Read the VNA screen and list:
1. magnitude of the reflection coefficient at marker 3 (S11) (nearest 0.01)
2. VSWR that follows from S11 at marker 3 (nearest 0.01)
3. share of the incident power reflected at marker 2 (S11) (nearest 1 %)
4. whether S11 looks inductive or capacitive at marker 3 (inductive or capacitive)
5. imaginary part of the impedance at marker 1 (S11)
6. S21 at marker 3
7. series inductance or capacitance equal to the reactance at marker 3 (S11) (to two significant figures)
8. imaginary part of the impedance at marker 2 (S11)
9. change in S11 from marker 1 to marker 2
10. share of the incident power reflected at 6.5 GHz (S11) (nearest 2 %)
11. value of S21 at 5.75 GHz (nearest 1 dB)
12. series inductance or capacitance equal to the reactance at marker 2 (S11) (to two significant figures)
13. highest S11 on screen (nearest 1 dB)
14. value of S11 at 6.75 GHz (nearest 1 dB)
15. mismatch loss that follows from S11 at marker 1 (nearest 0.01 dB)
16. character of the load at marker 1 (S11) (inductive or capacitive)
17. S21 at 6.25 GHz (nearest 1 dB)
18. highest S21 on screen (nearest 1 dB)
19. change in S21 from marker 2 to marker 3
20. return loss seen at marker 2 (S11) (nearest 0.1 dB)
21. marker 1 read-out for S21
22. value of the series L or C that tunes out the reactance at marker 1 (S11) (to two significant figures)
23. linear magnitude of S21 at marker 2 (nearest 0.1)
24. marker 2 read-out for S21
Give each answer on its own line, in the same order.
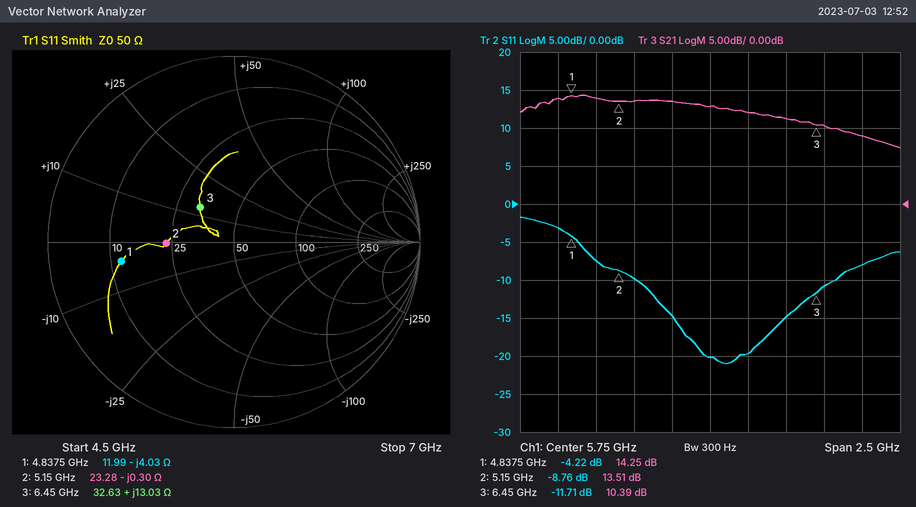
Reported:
0.26
1.70
13 %
inductive
-4.03 Ω
10.39 dB
320 pH
-0.30 Ω
-4.54 dB
8 %
13 dB
100 pF
-2 dB
-8 dB
2.07 dB
capacitive
11 dB
14 dB
-3.12 dB
8.8 dB
14.25 dB
130 pH
4.7
13.51 dB
